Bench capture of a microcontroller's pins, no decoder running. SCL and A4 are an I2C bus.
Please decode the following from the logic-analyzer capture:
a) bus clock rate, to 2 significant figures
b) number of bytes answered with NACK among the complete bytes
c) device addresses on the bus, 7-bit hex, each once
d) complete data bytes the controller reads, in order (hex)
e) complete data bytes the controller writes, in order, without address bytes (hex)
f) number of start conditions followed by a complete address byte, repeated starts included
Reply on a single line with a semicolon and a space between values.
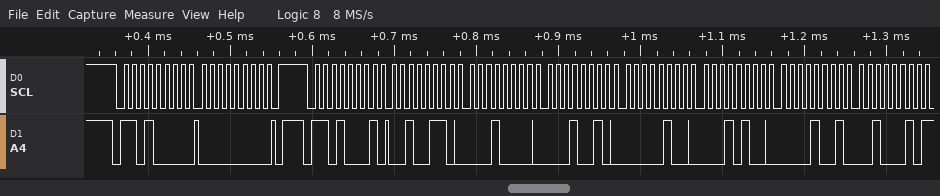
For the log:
100 kHz; 1; 0x68; 26 10 12 04 14 09 22; 00; 2
